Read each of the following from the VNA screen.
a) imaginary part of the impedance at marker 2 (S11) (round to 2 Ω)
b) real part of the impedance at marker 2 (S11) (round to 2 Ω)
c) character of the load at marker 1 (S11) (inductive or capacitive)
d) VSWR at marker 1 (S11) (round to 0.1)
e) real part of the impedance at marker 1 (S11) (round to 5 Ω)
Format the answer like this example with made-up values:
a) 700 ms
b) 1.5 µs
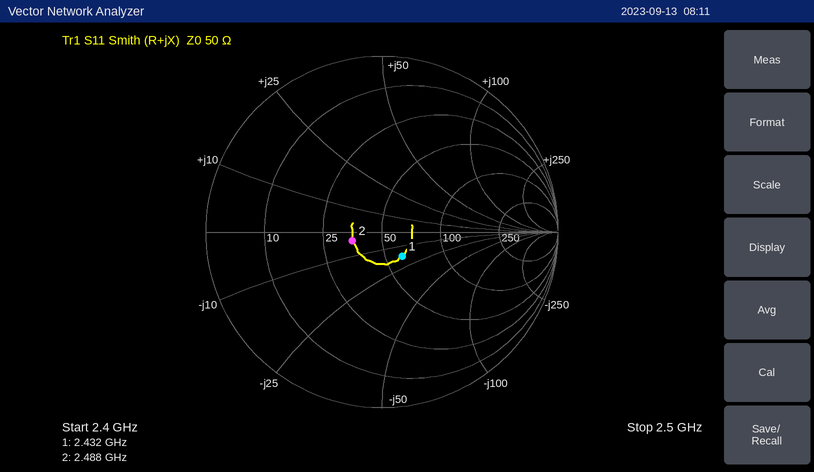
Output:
a) -4 Ω
b) 36 Ω
c) capacitive
d) 1.4
e) 60 Ω
